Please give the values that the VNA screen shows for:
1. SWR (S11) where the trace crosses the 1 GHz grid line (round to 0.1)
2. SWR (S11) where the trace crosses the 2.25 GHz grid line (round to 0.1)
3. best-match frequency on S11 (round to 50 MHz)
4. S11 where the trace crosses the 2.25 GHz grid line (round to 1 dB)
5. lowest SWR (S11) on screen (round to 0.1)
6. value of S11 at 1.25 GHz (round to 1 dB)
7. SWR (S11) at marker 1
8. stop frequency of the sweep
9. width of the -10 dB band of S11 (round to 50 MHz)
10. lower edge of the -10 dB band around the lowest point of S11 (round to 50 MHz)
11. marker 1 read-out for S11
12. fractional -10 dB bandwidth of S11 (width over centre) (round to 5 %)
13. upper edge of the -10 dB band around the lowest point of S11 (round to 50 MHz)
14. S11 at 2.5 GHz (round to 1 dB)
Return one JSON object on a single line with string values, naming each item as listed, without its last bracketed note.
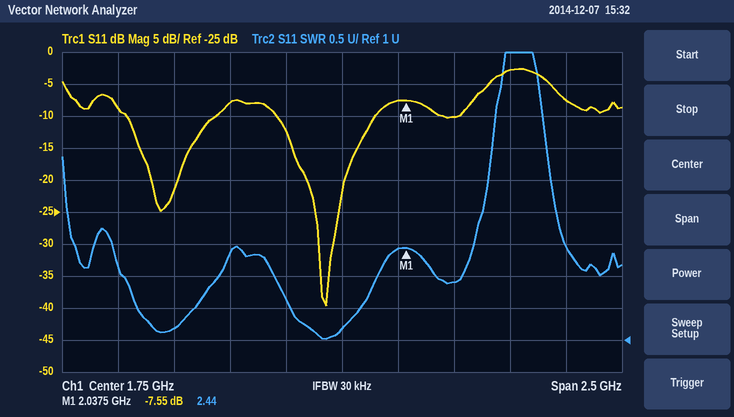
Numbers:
{"SWR (S11) where the trace crosses the 1 GHz grid line": "1.2", "SWR (S11) where the trace crosses the 2.25 GHz grid line": "1.9", "best-match frequency on S11": "1.70 GHz", "S11 where the trace crosses the 2.25 GHz grid line": "-10 dB", "lowest SWR (S11) on screen": "1.0", "value of S11 at 1.25 GHz": "-8 dB", "SWR (S11) at marker 1": "2.44", "stop frequency of the sweep": "3 GHz", "width of the -10 dB band of S11": "450 MHz", "lower edge of the -10 dB band around the lowest point of S11": "1.45 GHz", "marker 1 read-out for S11": "-7.55 dB", "fractional -10 dB bandwidth of S11 (width over centre)": "25 %", "upper edge of the -10 dB band around the lowest point of S11": "1.90 GHz", "S11 at 2.5 GHz": "-3 dB"}
